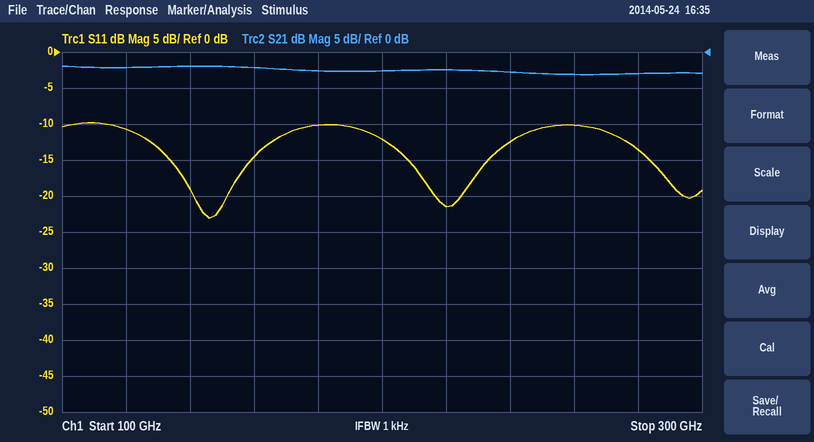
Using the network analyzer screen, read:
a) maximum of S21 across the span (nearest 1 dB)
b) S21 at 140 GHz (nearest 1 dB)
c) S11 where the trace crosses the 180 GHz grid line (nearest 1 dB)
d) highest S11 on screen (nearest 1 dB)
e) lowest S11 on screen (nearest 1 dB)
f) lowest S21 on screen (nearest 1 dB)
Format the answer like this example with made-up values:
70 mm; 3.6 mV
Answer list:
-2 dB; -2 dB; -10 dB; -10 dB; -23 dB; -3 dB
